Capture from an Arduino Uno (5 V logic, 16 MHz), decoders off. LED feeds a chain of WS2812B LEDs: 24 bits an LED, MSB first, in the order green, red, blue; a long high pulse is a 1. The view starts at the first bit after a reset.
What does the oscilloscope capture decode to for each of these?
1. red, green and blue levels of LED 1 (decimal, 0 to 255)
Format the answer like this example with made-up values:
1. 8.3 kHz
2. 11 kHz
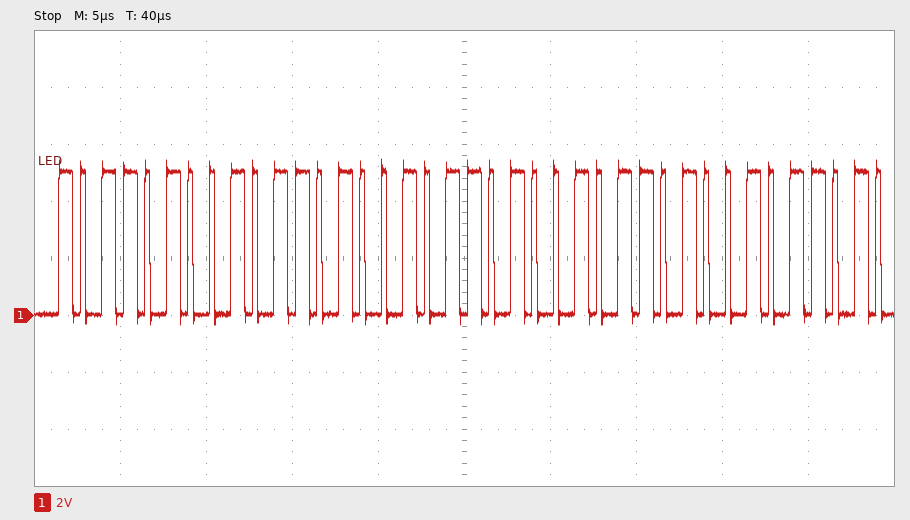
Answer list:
1. 180, 180, 180
